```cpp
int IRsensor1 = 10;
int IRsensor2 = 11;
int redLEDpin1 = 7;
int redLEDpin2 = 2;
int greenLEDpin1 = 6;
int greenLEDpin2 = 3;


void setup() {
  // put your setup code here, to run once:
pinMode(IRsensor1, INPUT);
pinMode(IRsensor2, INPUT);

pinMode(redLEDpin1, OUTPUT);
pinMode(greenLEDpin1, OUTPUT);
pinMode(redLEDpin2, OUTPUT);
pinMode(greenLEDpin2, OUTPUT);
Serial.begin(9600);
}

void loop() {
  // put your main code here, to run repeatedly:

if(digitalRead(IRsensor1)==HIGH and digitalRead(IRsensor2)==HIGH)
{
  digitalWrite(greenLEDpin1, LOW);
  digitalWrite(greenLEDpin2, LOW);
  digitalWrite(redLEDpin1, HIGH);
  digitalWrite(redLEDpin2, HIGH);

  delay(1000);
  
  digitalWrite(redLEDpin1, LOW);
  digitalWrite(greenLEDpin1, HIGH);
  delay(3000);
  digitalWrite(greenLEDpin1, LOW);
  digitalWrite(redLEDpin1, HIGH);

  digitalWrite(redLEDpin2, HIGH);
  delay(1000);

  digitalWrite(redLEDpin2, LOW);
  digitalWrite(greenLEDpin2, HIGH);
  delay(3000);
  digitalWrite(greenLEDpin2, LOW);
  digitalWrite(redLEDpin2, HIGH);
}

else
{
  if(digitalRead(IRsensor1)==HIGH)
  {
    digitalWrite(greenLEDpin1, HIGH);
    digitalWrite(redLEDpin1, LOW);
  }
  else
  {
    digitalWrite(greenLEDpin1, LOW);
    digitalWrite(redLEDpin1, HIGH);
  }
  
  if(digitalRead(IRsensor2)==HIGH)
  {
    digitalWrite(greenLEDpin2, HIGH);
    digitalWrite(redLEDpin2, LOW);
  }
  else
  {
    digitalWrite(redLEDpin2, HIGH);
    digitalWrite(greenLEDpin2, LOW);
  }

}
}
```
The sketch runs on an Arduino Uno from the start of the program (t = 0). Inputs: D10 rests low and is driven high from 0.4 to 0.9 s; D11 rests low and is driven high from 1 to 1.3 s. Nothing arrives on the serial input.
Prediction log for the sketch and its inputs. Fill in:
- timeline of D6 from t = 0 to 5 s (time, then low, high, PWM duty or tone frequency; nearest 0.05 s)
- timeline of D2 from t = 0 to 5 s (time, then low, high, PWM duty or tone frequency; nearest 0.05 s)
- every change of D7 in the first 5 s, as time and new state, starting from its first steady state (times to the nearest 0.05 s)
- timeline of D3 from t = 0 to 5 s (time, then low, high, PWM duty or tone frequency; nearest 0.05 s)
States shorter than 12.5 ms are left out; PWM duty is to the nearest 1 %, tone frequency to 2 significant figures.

0 s low; 0.4 s high; 0.9 s low
0 s high; 1 s low; 1.3 s high
0 s high; 0.4 s low; 0.9 s high
0 s low; 1 s high; 1.3 s low
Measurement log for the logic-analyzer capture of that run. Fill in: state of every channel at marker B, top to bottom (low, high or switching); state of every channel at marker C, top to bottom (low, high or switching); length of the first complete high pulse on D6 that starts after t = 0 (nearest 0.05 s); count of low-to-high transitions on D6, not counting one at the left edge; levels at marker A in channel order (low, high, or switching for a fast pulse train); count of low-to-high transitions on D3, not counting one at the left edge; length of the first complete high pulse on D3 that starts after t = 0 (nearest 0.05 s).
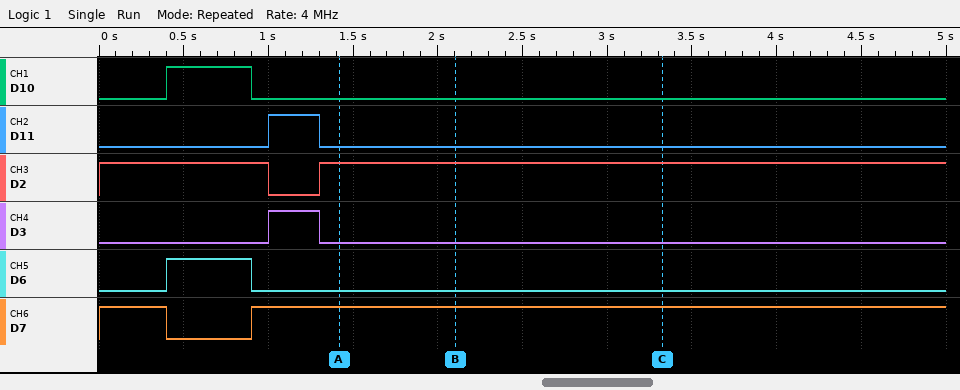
D10 low, D11 low, D2 high, D3 low, D6 low, D7 high
D10 low, D11 low, D2 high, D3 low, D6 low, D7 high
0.50 s
1
D10 low, D11 low, D2 high, D3 low, D6 low, D7 high
1
0.30 s
